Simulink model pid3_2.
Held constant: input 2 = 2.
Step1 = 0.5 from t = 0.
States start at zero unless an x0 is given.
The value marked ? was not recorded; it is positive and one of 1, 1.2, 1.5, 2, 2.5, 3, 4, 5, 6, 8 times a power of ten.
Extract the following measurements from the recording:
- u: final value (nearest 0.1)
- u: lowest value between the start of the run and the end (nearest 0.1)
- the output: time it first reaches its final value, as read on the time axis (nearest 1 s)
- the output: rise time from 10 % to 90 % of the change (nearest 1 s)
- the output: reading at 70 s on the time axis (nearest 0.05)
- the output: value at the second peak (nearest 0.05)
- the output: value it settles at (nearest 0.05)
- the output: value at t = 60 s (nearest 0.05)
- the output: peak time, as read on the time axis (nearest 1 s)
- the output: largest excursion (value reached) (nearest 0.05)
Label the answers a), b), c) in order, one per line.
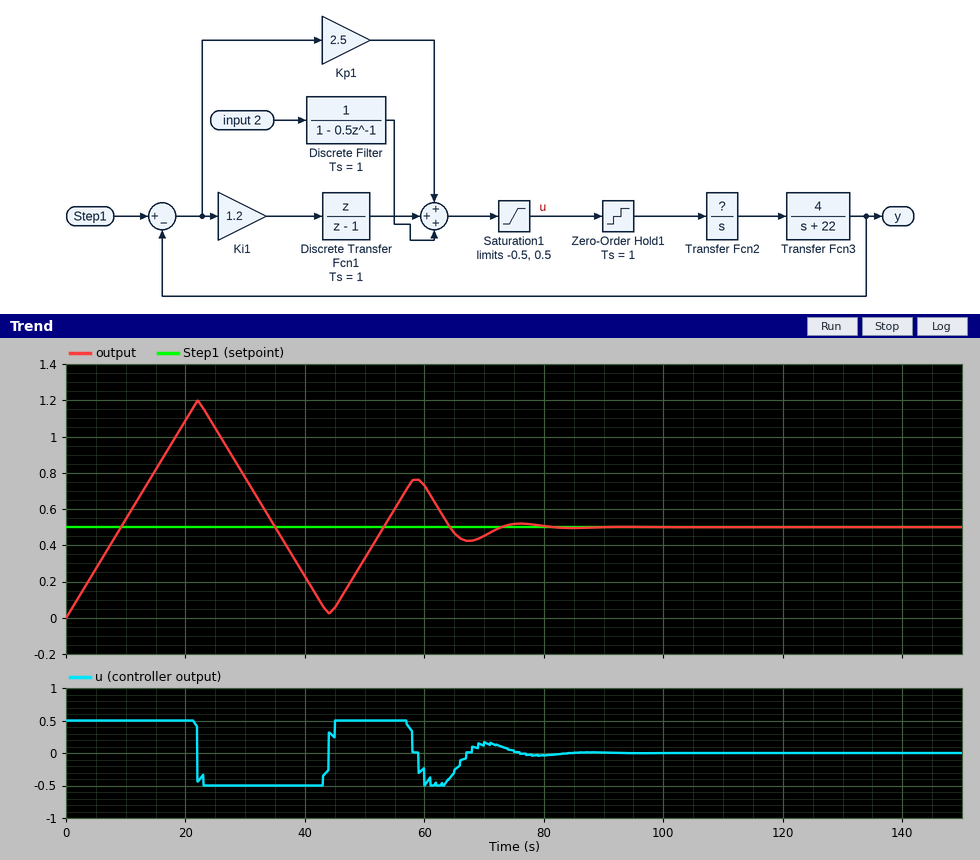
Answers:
a) 0.0
b) -0.5
c) 9 s
d) 7 s
e) 0.45
f) 0.75
g) 0.50
h) 0.75
i) 22 s
j) 1.20
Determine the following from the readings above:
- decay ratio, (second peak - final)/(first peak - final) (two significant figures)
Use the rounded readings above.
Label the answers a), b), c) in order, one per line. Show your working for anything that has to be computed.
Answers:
a) (0.75 - 0.5) / (1.2 - 0.5) = 0.36
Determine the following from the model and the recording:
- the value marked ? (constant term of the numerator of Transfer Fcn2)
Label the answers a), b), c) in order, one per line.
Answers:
a) 0.6
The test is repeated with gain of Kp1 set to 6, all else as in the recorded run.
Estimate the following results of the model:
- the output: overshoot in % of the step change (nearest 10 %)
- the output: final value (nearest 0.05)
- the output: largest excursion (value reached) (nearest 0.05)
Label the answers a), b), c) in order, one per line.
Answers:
a) 120 %
b) 0.50
c) 1.10
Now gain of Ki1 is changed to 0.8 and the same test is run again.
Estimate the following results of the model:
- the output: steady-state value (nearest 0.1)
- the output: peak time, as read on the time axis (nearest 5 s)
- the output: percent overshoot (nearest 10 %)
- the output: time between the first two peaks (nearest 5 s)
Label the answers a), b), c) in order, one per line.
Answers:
a) 0.5
b) 25 s
c) 150 %
d) 35 s
